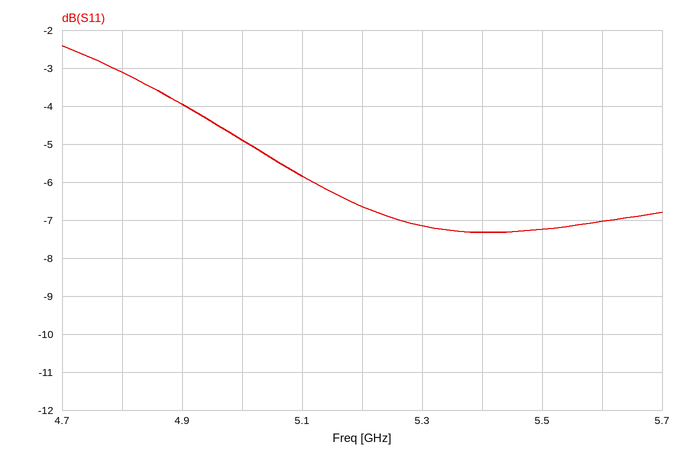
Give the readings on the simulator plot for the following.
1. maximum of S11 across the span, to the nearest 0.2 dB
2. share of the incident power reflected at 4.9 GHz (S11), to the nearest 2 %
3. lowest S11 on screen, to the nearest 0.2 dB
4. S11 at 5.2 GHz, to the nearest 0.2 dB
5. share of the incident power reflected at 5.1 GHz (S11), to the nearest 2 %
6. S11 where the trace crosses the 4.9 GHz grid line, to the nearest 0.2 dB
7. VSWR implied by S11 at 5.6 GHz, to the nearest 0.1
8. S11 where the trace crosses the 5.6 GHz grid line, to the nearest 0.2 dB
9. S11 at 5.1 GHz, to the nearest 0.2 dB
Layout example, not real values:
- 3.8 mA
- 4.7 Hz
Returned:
- -2.4 dB
- 40 %
- -7.4 dB
- -6.6 dB
- 26 %
- -4.0 dB
- 2.6
- -7.0 dB
- -5.8 dB
